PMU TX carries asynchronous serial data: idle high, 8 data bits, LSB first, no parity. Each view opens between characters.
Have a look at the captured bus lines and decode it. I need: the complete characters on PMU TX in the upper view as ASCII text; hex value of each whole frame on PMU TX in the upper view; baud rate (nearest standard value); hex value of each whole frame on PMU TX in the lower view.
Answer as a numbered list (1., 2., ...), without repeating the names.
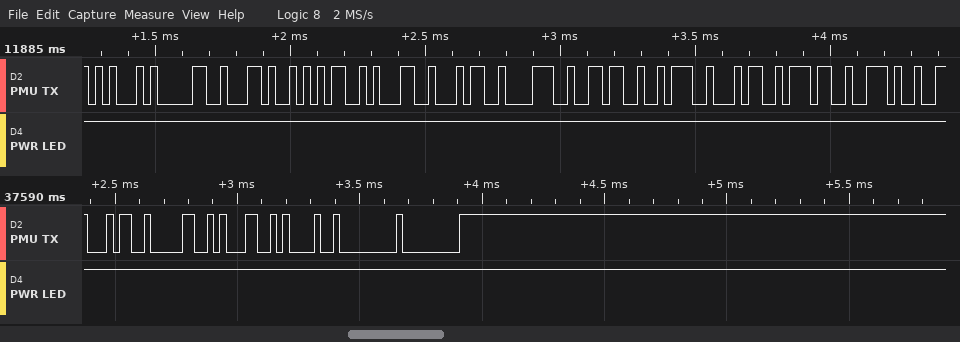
1. "E0,51486:47."
2. 45, 30, 2C, 35, 31, 34, 38, 36, 3A, 34, 37, 2E
3. 38400 baud
4. 34, 30, 31, 21, 00, 00
